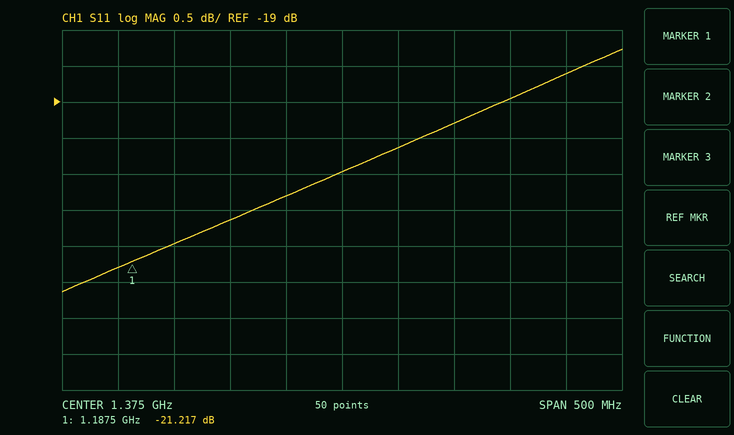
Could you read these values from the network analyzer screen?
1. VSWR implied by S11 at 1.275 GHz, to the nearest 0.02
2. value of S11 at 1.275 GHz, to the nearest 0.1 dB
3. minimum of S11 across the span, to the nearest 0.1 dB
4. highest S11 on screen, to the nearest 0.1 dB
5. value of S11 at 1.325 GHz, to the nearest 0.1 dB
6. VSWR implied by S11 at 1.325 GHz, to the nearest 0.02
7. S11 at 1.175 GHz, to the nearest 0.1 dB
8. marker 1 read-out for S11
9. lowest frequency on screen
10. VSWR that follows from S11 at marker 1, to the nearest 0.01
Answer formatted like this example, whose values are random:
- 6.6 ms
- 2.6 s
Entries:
- 1.20
- -20.6 dB
- -21.6 dB
- -18.3 dB
- -20.3 dB
- 1.22
- -21.3 dB
- -21.217 dB
- 1.125 GHz
- 1.19
